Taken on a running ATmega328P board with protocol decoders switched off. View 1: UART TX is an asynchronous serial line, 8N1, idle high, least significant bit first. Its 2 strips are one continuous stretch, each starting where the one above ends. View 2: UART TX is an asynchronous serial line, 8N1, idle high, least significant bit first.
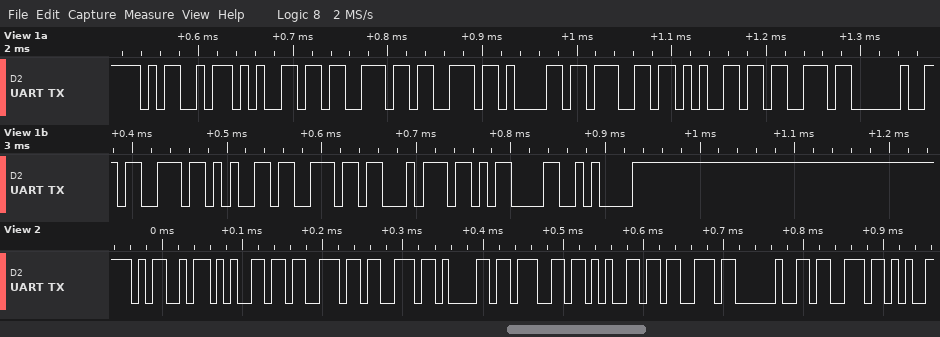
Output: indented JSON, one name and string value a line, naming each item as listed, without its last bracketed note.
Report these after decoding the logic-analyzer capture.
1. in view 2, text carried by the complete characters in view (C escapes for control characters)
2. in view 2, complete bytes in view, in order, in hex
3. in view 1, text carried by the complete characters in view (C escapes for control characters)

{
  "in view 2, text carried by the complete characters in view": "\"Messages s\"",
  "in view 2, complete bytes in view, in order, in hex": "0x4D 0x65 0x73 0x73 0x61 0x67 0x65 0x73 0x20 0x73",
  "in view 1, text carried by the complete characters in view": "\"Messages sent\\r\\n\""
}
